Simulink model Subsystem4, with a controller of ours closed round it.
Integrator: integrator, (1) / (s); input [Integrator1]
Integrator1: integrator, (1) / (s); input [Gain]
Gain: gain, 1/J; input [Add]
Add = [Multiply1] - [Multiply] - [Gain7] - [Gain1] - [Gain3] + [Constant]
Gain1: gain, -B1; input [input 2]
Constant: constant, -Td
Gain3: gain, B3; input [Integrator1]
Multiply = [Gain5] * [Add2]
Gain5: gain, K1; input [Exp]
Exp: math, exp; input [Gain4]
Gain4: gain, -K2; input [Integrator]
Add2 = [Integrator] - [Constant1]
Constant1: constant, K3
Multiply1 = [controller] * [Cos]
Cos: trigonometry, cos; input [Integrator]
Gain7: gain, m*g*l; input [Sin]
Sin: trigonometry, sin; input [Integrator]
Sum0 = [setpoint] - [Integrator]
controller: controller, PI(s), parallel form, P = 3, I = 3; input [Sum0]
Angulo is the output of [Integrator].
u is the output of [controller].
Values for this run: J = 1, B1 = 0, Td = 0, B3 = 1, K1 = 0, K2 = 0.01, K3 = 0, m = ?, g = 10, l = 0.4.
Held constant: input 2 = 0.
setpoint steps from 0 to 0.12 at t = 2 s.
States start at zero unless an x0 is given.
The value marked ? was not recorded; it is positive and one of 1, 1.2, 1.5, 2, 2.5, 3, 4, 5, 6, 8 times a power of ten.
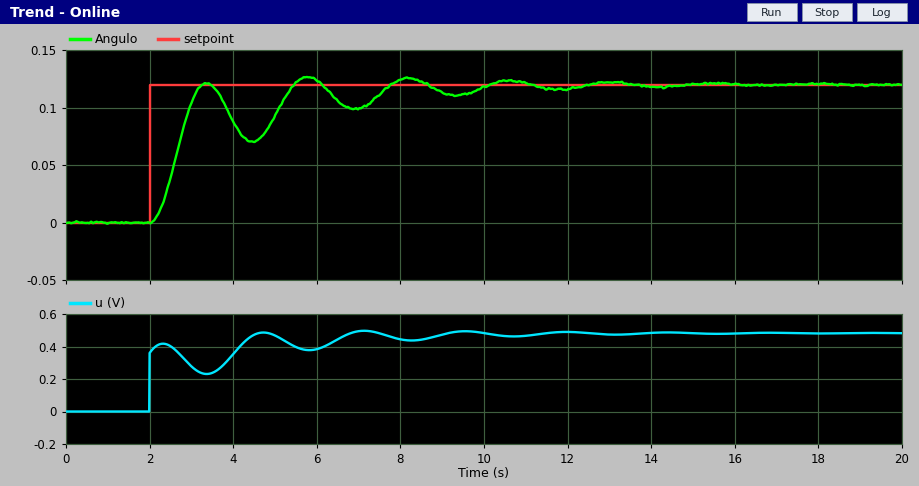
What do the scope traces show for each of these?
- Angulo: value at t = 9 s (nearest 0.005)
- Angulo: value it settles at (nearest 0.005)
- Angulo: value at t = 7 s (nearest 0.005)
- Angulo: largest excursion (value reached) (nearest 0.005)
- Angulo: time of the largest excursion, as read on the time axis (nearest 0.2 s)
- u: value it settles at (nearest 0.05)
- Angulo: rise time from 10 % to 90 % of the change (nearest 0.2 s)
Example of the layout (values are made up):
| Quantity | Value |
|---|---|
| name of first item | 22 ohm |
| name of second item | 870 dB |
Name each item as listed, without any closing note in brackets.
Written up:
| Quantity | Value |
|---|---|
| Angulo: value at t = 9 s | 0.115 |
| Angulo: value it settles at | 0.120 |
| Angulo: value at t = 7 s | 0.100 |
| Angulo: largest excursion (value reached) | 0.125 |
| Angulo: time of the largest excursion, as read on the time axis | 5.8 s |
| u: value it settles at | 0.50 |
| Angulo: rise time from 10 % to 90 % of the change | 0.8 s |
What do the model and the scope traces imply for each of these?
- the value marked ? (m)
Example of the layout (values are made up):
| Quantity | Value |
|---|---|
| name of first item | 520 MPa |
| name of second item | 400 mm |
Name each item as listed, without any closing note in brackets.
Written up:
| Quantity | Value |
|---|---|
| the value marked ? | 1 |
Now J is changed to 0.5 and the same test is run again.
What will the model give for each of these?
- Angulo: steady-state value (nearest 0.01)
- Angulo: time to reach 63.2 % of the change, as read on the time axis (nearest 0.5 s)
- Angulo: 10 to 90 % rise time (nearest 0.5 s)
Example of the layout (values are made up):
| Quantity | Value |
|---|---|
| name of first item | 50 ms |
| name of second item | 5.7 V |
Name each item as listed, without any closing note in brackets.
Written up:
| Quantity | Value |
|---|---|
| Angulo: steady-state value | 0.12 |
| Angulo: time to reach 63.2 % of the change, as read on the time axis | 2.5 s |
| Angulo: 10 to 90 % rise time | 4.0 s |
